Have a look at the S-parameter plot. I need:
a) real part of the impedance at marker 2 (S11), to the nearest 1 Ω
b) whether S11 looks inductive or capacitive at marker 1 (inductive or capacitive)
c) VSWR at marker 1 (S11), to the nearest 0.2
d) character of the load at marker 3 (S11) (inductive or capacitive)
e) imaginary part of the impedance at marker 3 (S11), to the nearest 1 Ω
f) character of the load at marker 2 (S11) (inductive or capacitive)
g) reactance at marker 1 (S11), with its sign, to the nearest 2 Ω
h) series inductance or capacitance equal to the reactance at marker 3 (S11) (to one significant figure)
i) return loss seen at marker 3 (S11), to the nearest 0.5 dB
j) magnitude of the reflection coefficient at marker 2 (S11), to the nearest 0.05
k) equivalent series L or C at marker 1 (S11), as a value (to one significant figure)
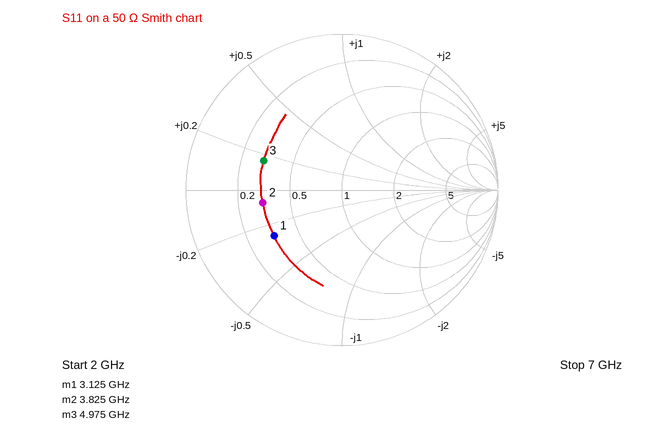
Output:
16 Ω
capacitive
3.2
inductive
+8 Ω
capacitive
-14 Ω
300 pH
5.5 dB
0.50
4 pF
